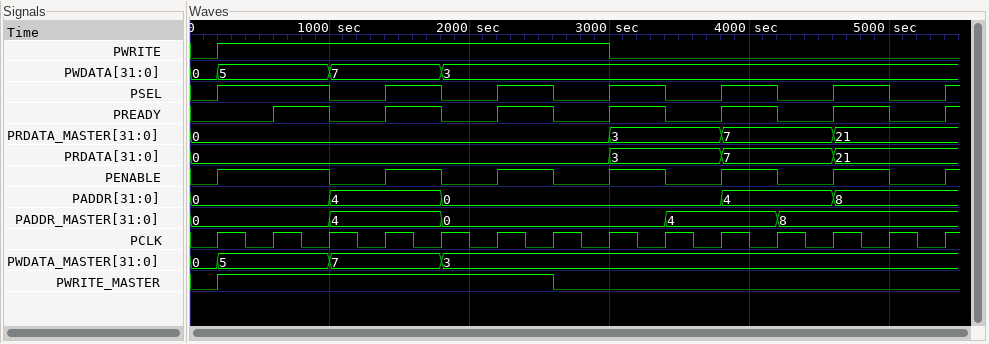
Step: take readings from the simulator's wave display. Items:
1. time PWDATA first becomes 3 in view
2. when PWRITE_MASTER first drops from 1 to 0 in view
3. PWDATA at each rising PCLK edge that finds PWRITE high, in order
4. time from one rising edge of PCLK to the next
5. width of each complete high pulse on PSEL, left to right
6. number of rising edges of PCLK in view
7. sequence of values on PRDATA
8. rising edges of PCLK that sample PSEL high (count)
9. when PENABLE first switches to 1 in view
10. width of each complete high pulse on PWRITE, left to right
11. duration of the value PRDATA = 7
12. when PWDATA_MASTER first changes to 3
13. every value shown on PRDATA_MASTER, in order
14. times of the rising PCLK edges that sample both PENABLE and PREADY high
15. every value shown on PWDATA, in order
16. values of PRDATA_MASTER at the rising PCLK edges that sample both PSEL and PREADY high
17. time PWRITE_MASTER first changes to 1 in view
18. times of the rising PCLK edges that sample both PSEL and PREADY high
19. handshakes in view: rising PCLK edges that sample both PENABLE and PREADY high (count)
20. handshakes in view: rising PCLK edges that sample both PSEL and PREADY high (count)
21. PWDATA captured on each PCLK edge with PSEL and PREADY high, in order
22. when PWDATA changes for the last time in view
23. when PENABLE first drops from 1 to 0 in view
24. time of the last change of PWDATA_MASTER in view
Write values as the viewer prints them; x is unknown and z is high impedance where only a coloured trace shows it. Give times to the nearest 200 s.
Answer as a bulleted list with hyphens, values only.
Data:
- 1800 s
- 2600 s
- 5, 5, 7, 7, 3, 3, 3
- 400 s
- 800 s, 400 s, 400 s, 400 s, 400 s, 400 s
- 14
- 0, 3, 7, 21
- 7
- 200 s
- 2800 s
- 800 s
- 1800 s
- 0, 3, 7, 21
- 1000 s, 1800 s, 2600 s, 3400 s, 4200 s, 5000 s
- 0, 5, 7, 3
- 0, 0, 0, 3, 7, 21
- 200 s
- 1000 s, 1800 s, 2600 s, 3400 s, 4200 s, 5000 s
- 6
- 6
- 5, 7, 3, 3, 3, 3
- 1800 s
- 1000 s
- 1800 s
